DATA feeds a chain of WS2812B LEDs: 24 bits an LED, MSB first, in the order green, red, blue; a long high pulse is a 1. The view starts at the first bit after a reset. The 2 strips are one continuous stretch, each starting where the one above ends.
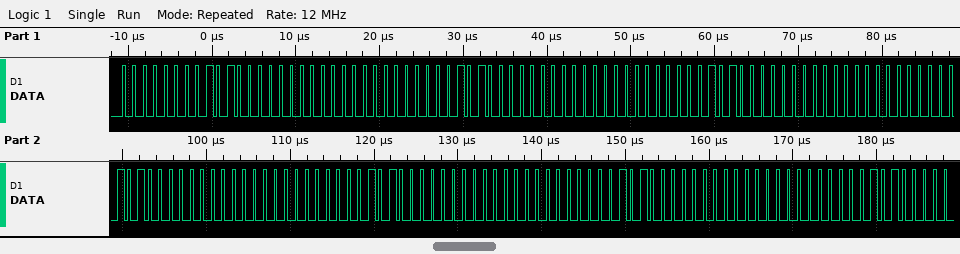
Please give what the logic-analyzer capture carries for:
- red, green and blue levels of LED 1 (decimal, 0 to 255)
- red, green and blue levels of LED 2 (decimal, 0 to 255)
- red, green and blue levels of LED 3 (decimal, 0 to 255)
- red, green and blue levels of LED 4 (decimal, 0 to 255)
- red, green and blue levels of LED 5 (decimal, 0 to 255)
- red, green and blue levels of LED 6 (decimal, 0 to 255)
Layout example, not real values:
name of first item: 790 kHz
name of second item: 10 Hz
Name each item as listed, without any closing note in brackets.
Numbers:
red, green and blue levels of LED 1: 160, 0, 0
red, green and blue levels of LED 2: 160, 0, 0
red, green and blue levels of LED 3: 160, 0, 0
red, green and blue levels of LED 4: 160, 0, 0
red, green and blue levels of LED 5: 160, 0, 0
red, green and blue levels of LED 6: 160, 0, 0
